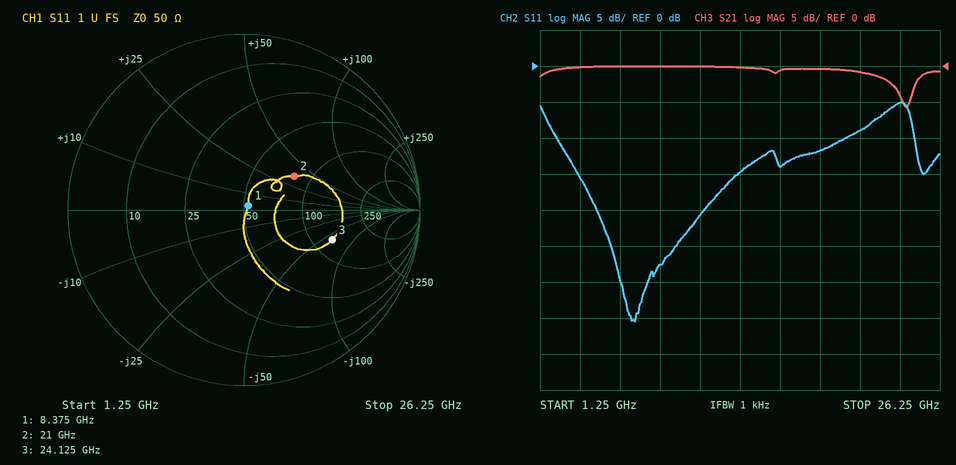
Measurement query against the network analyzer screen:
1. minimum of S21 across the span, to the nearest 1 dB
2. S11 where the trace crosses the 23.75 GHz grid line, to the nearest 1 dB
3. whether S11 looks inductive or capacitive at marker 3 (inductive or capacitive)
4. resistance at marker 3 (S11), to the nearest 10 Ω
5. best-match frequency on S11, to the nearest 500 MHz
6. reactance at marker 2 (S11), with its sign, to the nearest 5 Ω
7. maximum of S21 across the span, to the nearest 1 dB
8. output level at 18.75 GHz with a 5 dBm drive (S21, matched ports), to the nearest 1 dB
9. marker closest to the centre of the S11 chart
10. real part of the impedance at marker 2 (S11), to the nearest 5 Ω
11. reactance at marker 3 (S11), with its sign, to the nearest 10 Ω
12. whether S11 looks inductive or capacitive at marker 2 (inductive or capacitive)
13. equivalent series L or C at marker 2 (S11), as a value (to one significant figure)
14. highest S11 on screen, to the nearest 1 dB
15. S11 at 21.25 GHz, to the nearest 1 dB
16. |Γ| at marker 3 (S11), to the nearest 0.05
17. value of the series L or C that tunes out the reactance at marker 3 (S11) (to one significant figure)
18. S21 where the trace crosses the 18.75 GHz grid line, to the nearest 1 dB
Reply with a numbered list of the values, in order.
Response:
1. -6 dB
2. -5 dB
3. capacitive
4. 130 Ω
5. 7.0 GHz
6. +35 Ω
7. 0 dB
8. 5 dBm
9. marker 1
10. 80 Ω
11. -60 Ω
12. inductive
13. 300 pH
14. -5 dB
15. -9 dB
16. 0.55
17. 400 pH
18. 0 dB
